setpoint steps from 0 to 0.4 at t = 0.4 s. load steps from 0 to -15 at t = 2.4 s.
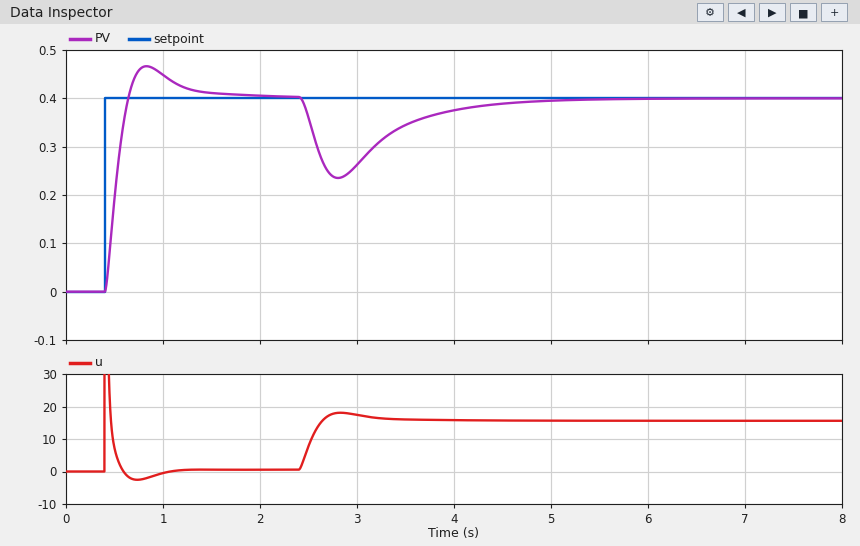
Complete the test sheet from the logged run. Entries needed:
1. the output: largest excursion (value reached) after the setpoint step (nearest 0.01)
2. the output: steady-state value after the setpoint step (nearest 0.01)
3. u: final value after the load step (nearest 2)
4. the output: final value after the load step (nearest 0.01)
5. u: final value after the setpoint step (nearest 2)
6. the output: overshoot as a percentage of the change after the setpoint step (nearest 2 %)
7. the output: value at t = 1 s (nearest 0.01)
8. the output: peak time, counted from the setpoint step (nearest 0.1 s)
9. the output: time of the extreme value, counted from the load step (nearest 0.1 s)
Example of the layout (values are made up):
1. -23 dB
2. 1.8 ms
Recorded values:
1. 0.47
2. 0.40
3. 16
4. 0.40
5. 0
6. 16 %
7. 0.45
8. 0.4 s
9. 0.4 s
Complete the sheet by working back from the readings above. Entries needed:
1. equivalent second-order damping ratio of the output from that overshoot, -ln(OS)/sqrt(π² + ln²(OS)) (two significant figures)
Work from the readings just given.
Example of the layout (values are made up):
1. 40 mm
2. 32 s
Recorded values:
1. 0.50
